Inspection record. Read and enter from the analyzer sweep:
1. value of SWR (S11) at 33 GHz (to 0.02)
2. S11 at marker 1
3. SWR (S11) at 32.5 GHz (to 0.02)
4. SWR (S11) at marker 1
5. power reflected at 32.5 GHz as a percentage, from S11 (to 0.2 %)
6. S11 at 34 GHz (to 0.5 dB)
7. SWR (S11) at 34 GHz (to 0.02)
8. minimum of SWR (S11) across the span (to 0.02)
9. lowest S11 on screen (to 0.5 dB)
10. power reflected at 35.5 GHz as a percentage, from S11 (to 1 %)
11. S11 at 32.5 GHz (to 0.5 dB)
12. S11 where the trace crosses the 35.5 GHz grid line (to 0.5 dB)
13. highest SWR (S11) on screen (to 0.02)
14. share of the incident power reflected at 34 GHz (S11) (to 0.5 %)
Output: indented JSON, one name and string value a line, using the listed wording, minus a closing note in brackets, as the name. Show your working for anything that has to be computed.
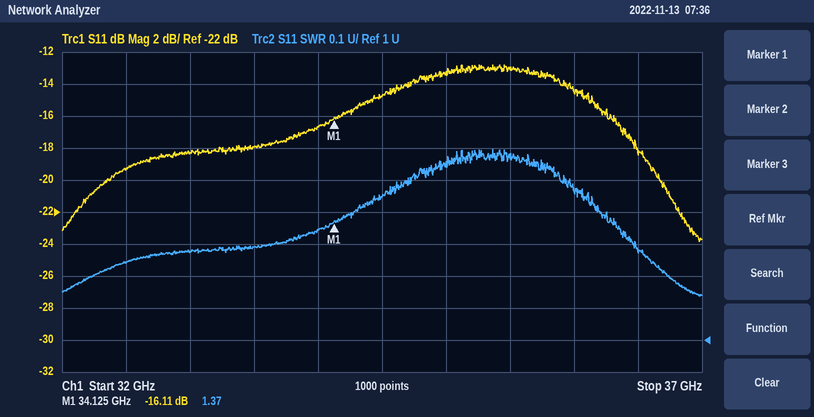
{
  "value of SWR (S11) at 33 GHz": "1.28",
  "S11 at marker 1": "-16.11 dB",
  "SWR (S11) at 32.5 GHz": "1.24",
  "SWR (S11) at marker 1": "1.37",
  "power reflected at 32.5 GHz as a percentage, from S11": "10^(-19.5/10) ≈ 1.12 %, so 1.2 % to the nearest 0.2 %",
  "S11 at 34 GHz": "-16.5 dB",
  "SWR (S11) at 34 GHz": "1.34",
  "minimum of SWR (S11) across the span": "1.14",
  "lowest S11 on screen": "-24.0 dB",
  "power reflected at 35.5 GHz as a percentage, from S11": "10^(-13/10) ≈ 5 %",
  "S11 at 32.5 GHz": "-19.5 dB",
  "S11 where the trace crosses the 35.5 GHz grid line": "-13.0 dB",
  "highest SWR (S11) on screen": "1.60",
  "share of the incident power reflected at 34 GHz (S11)": "10^(-16.5/10) ≈ 2.24 %, so 2.0 % to the nearest 0.5 %"
}
